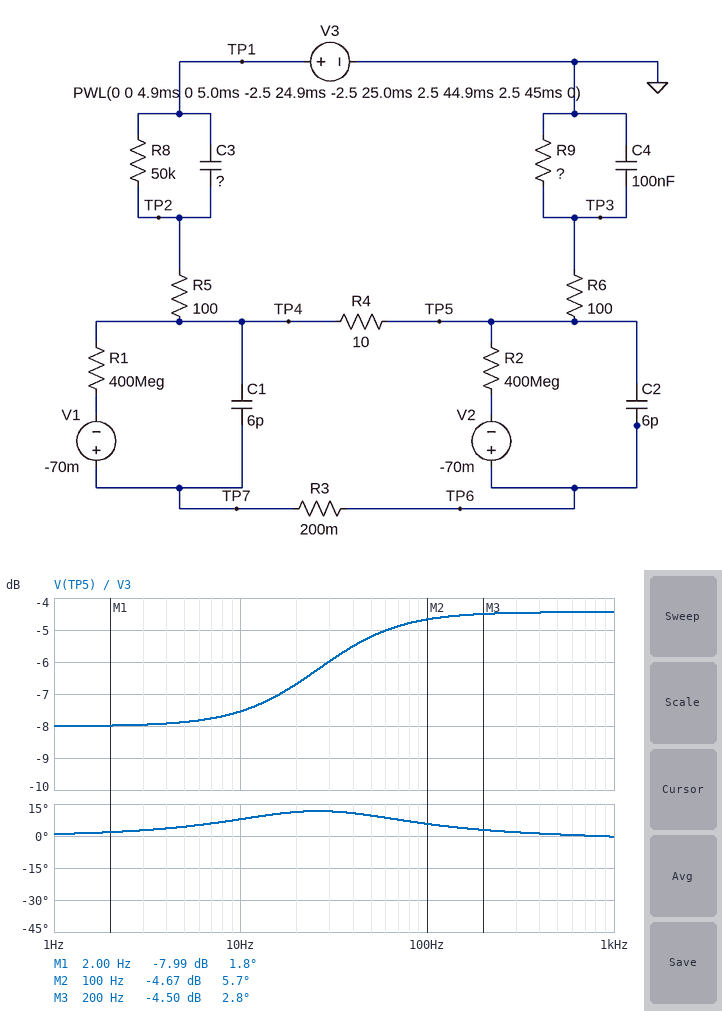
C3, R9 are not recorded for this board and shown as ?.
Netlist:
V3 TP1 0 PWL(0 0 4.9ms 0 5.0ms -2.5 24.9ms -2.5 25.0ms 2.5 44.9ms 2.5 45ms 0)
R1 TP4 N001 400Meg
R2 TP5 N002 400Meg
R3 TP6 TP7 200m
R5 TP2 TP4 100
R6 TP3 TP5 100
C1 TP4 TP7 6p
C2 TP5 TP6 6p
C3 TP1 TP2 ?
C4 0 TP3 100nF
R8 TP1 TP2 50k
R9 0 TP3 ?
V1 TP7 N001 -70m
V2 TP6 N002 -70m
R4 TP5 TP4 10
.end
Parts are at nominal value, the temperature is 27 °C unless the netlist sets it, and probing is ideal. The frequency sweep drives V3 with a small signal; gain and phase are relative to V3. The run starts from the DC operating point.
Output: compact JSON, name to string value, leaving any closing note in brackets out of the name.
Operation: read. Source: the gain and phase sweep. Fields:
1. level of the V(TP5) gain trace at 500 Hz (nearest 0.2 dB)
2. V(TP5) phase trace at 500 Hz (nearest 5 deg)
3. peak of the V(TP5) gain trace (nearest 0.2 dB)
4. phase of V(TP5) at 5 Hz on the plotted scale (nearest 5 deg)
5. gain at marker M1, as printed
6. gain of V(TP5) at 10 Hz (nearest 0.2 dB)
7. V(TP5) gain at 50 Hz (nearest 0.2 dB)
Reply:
{"level of the V(TP5) gain trace at 500 Hz": "-4.4 dB", "V(TP5) phase trace at 500 Hz": "0 deg", "peak of the V(TP5) gain trace": "-4.4 dB", "phase of V(TP5) at 5 Hz on the plotted scale": "5 deg", "gain at marker M1, as printed": "-7.99 dB", "gain of V(TP5) at 10 Hz": "-7.6 dB", "V(TP5) gain at 50 Hz": "-5.2 dB"}
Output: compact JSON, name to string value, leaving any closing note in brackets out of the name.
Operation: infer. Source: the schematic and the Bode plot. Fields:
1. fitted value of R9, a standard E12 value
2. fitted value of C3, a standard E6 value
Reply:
{"fitted value of R9, a standard E12 value": "33 kΩ", "fitted value of C3, a standard E6 value": "150 nF"}
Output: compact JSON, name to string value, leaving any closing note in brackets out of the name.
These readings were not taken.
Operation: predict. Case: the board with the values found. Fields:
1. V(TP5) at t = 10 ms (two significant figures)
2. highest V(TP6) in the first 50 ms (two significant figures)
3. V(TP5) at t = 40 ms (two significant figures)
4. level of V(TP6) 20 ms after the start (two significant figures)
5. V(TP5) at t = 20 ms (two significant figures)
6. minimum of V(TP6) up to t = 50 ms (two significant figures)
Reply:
{"V(TP5) at t = 10 ms": "-1.2 V", "highest V(TP6) in the first 50 ms": "1.9 V", "V(TP5) at t = 40 ms": "1.0 V", "level of V(TP6) 20 ms after the start": "-1.1 V", "V(TP5) at t = 20 ms": "-1.0 V", "minimum of V(TP6) up to t = 50 ms": "-1.6 V"}
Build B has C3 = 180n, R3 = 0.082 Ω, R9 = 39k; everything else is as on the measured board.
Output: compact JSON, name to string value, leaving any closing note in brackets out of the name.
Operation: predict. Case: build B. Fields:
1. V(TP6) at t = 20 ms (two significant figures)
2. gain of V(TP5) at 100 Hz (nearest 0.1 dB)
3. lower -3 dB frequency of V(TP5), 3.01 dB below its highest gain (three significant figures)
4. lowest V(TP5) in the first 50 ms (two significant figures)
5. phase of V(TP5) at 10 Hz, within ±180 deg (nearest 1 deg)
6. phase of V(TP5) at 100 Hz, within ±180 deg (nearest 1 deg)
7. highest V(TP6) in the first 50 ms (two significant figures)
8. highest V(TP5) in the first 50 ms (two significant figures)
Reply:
{"V(TP6) at t = 20 ms": "-1.2 V", "gain of V(TP5) at 100 Hz": "-4.0 dB", "lower -3 dB frequency of V(TP5), 3.01 dB below its highest gain": "6.75 Hz", "lowest V(TP5) in the first 50 ms": "-1.6 V", "phase of V(TP5) at 10 Hz, within ±180 deg": "8 deg", "phase of V(TP5) at 100 Hz, within ±180 deg": "4 deg", "highest V(TP6) in the first 50 ms": "2.0 V", "highest V(TP5) in the first 50 ms": "2.1 V"}
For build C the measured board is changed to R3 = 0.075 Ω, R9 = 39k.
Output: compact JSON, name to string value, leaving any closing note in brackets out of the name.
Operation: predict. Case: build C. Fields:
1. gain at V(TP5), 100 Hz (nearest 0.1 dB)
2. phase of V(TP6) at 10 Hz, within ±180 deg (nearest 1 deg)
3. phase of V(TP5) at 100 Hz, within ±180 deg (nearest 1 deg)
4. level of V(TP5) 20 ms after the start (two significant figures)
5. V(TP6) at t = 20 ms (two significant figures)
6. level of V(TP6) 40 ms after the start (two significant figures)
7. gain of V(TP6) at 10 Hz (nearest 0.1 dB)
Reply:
{"gain at V(TP5), 100 Hz": "-4.6 dB", "phase of V(TP6) at 10 Hz, within ±180 deg": "6 deg", "phase of V(TP5) at 100 Hz, within ±180 deg": "4 deg", "level of V(TP5) 20 ms after the start": "-1.1 V", "V(TP6) at t = 20 ms": "-1.2 V", "level of V(TP6) 40 ms after the start": "1.1 V", "gain of V(TP6) at 10 Hz": "-6.8 dB"}
